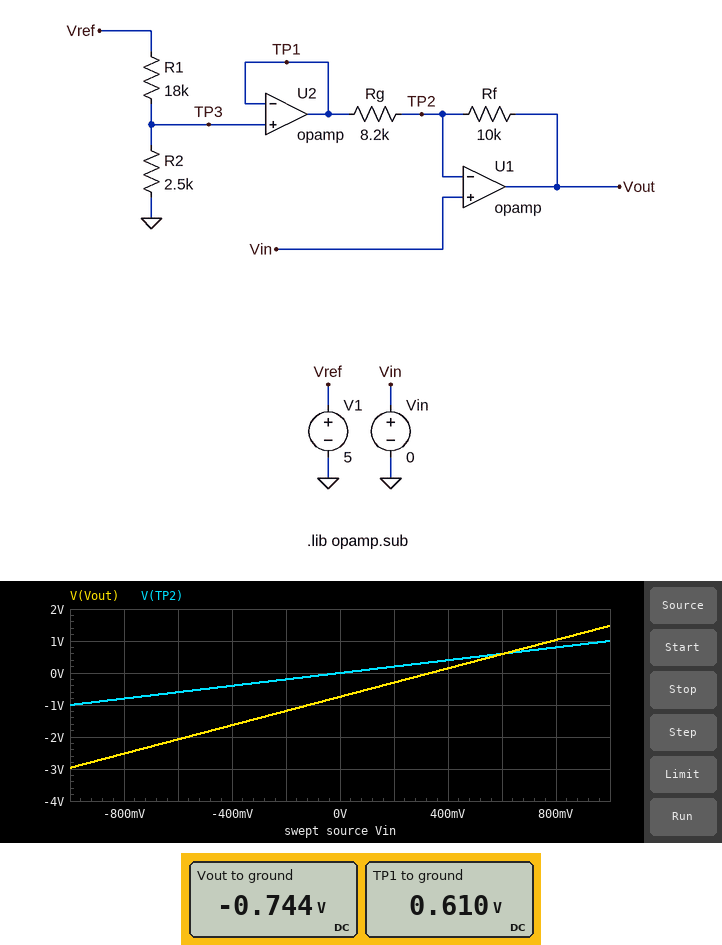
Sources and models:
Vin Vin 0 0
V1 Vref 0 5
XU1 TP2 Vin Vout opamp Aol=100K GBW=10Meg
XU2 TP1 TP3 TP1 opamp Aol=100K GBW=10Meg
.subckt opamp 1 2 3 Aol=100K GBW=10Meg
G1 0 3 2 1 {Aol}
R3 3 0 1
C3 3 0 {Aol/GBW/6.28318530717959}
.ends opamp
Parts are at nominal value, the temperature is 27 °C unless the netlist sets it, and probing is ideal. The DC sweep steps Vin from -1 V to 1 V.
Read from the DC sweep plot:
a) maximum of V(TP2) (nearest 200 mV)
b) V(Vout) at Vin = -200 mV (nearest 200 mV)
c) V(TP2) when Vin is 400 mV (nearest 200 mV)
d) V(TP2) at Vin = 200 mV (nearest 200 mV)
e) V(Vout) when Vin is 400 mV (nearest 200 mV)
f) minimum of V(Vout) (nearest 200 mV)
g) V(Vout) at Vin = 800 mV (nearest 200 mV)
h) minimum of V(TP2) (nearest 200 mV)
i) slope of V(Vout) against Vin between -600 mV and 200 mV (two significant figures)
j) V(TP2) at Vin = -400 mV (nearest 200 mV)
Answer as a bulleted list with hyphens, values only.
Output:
- 1.0 V
- -1.2 V
- 400 mV
- 200 mV
- 200 mV
- -3.0 V
- 1.0 V
- -1.0 V
- 2.2 V/V
- -400 mV
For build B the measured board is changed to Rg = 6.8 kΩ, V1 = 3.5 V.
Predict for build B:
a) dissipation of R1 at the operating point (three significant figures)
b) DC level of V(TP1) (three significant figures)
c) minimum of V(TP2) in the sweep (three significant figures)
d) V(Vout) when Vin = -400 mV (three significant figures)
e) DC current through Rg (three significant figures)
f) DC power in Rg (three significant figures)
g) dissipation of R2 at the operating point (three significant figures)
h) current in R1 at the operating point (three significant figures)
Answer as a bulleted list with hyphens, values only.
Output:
- 525 µW
- 427 mV
- -1.00 V
- -1.62 V
- 62.8 µA
- 26.8 µW
- 72.9 µW
- 171 µA
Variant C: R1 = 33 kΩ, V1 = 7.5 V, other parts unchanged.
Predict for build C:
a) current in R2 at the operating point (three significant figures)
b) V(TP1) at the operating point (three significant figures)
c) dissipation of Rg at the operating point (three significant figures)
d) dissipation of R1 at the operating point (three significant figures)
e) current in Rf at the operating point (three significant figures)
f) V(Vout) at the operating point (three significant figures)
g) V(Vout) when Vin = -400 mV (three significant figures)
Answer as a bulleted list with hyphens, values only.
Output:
- 211 µA
- 528 mV
- 34.0 µW
- 1.47 mW
- 64.4 µA
- -644 mV
- -1.53 V
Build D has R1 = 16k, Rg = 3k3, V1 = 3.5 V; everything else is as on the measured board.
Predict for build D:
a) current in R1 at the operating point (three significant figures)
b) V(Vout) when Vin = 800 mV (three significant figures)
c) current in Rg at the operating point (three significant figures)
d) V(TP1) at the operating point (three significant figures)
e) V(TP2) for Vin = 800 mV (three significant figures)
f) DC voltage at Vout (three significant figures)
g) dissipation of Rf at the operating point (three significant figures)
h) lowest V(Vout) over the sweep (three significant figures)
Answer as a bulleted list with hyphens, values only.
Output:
- 189 µA
- 1.79 V
- 143 µA
- 473 mV
- 800 mV
- -1.43 V
- 205 µW
- -5.46 V
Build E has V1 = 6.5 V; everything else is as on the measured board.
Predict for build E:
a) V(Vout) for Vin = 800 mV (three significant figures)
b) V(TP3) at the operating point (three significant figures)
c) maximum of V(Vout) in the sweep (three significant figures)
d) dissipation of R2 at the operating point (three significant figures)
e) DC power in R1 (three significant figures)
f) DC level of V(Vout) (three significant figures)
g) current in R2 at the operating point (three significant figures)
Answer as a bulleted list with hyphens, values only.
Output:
- 809 mV
- 793 mV
- 1.25 V
- 251 µW
- 1.81 mW
- -967 mV
- 317 µA
